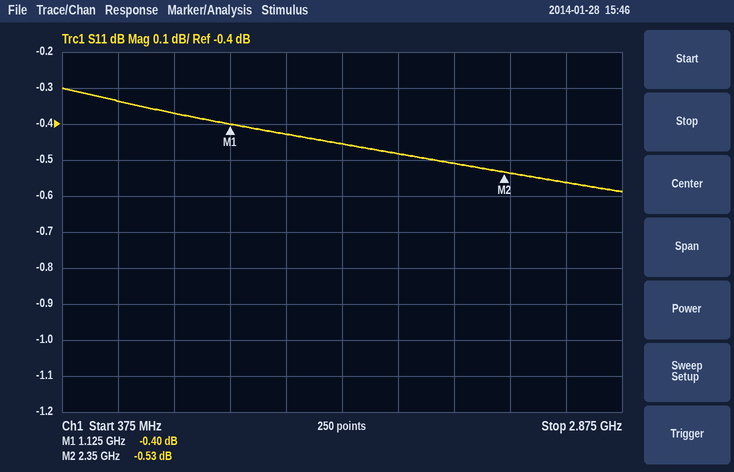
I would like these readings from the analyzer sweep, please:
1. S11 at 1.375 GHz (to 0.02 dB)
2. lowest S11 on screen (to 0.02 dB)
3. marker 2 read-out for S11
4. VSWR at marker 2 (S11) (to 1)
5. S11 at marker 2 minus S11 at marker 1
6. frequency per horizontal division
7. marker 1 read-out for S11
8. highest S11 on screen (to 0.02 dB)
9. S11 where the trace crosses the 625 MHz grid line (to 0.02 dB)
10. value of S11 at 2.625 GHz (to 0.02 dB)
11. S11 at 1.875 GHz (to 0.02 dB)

-0.42 dB
-0.58 dB
-0.53 dB
33
-0.13 dB
250 MHz
-0.40 dB
-0.30 dB
-0.34 dB
-0.56 dB
-0.48 dB
